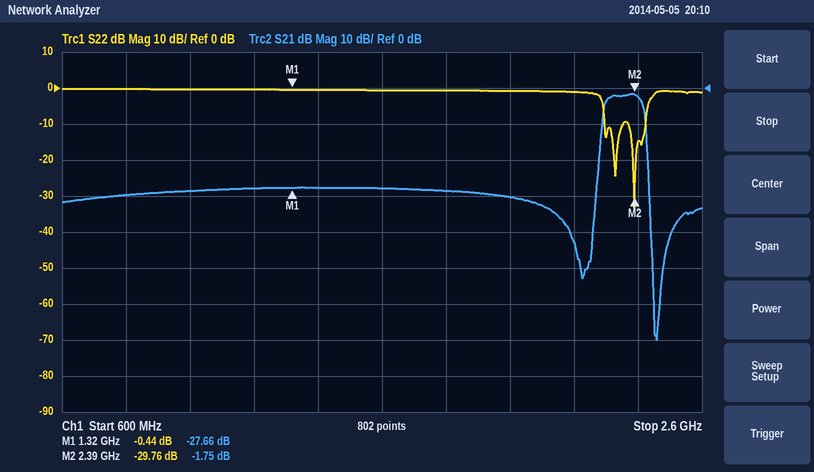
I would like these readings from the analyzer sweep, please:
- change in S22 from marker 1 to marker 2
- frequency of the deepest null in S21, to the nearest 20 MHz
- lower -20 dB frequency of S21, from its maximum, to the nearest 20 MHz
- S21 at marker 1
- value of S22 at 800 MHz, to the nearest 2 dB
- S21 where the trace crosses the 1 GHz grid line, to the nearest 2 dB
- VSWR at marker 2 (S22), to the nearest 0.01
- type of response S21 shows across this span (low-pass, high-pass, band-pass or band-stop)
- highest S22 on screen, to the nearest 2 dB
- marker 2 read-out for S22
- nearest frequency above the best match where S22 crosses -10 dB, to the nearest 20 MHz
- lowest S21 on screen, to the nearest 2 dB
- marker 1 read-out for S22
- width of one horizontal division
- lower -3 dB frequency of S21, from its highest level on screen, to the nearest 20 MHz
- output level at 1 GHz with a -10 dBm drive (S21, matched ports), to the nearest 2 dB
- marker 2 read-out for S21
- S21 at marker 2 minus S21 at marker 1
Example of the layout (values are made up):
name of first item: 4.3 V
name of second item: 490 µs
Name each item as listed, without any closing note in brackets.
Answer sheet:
change in S22 from marker 1 to marker 2: -29.32 dB
frequency of the deepest null in S21, to the nearest 20 MHz: 2.46 GHz
lower -20 dB frequency of S21, from its maximum, to the nearest 20 MHz: 2.28 GHz
S21 at marker 1: -27.66 dB
value of S22 at 800 MHz, to the nearest 2 dB: 0 dB
S21 where the trace crosses the 1 GHz grid line, to the nearest 2 dB: -28 dB
VSWR at marker 2 (S22), to the nearest 0.01: 1.07
type of response S21 shows across this span: band-pass
highest S22 on screen, to the nearest 2 dB: 0 dB
marker 2 read-out for S22: -29.76 dB
nearest frequency above the best match where S22 crosses -10 dB, to the nearest 20 MHz: 2.42 GHz
lowest S21 on screen, to the nearest 2 dB: -70 dB
marker 1 read-out for S22: -0.44 dB
width of one horizontal division: 200 MHz
lower -3 dB frequency of S21, from its highest level on screen, to the nearest 20 MHz: 2.30 GHz
output level at 1 GHz with a -10 dBm drive (S21, matched ports), to the nearest 2 dB: -38 dBm
marker 2 read-out for S21: -1.75 dB
S21 at marker 2 minus S21 at marker 1: 25.91 dB
